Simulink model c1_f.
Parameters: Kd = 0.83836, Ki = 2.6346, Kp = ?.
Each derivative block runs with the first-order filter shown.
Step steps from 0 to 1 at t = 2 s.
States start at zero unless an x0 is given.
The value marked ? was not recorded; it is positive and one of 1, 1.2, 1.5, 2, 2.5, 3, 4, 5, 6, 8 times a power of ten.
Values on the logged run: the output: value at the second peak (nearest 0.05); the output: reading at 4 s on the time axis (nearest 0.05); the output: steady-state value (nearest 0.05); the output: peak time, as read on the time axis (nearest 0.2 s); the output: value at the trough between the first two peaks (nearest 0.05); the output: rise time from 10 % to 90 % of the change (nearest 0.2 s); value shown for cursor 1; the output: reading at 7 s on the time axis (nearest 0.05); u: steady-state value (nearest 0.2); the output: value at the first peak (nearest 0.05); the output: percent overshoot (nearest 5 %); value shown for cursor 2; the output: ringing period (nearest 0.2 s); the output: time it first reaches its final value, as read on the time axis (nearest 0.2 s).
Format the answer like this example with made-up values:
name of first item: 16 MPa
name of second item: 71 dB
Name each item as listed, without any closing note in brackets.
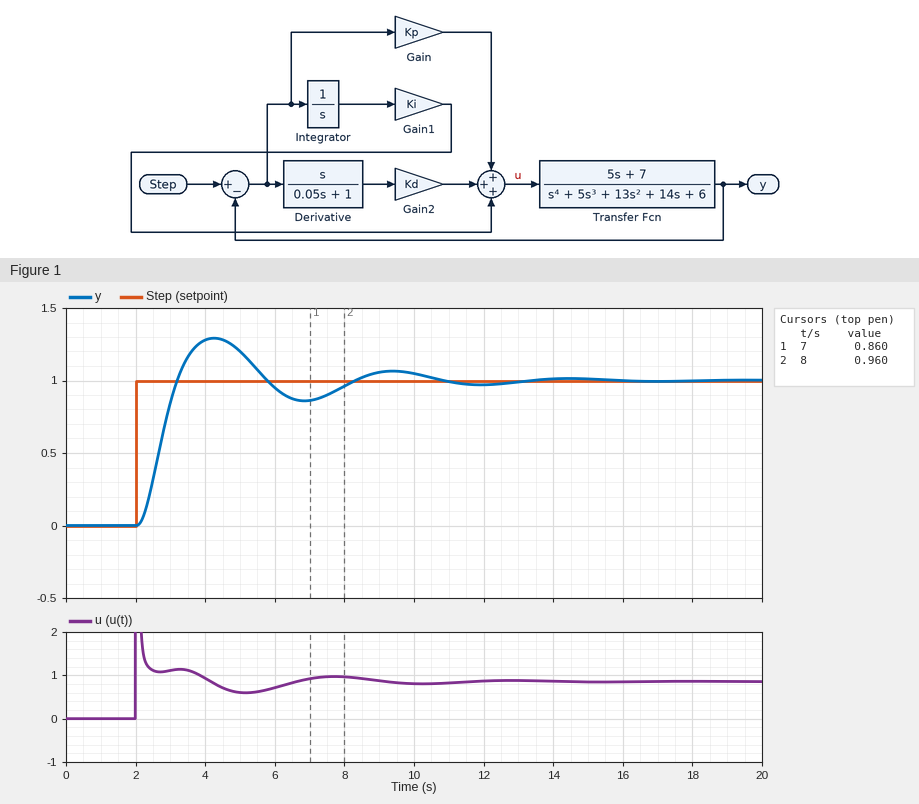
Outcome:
the output: value at the second peak: 1.05
the output: reading at 4 s on the time axis: 1.30
the output: steady-state value: 1.00
the output: peak time, as read on the time axis: 4.2 s
the output: value at the trough between the first two peaks: 0.85
the output: rise time from 10 % to 90 % of the change: 0.8 s
value shown for cursor 1: 0.860
the output: reading at 7 s on the time axis: 0.85
u: steady-state value: 0.8
the output: value at the first peak: 1.30
the output: percent overshoot: 30 %
value shown for cursor 2: 0.960
the output: ringing period: 5.2 s
the output: time it first reaches its final value, as read on the time axis: 3.2 s
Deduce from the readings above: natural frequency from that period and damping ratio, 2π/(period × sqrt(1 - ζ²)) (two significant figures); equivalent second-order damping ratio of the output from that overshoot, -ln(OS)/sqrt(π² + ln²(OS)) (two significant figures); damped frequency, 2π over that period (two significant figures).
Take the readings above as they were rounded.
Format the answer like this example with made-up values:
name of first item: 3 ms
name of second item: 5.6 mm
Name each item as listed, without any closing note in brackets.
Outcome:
natural frequency from that period and damping ratio, 2π/(period × sqrt(1 - ζ²)): 1.3 rad/s
equivalent second-order damping ratio of the output from that overshoot, -ln(OS)/sqrt(π² + ln²(OS)): 0.36
damped frequency, 2π over that period: 1.2 rad/s
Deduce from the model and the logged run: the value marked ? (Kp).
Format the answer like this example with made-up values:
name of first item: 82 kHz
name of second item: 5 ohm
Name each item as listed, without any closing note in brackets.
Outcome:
the value marked ?: 1.2
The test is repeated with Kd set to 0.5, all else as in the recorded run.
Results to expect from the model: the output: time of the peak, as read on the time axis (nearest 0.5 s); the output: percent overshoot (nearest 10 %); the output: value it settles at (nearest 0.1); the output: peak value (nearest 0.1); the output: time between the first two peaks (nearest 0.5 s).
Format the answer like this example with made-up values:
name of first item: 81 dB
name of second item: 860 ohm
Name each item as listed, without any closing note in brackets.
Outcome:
the output: time of the peak, as read on the time axis: 4.0 s
the output: percent overshoot: 50 %
the output: value it settles at: 1.0
the output: peak value: 1.5
the output: time between the first two peaks: 4.5 s
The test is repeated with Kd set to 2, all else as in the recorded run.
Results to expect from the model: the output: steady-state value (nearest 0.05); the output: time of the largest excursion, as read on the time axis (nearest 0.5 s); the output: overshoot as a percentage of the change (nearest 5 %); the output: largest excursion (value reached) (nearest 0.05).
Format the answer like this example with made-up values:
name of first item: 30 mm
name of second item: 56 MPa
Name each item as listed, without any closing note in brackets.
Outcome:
the output: steady-state value: 1.00
the output: time of the largest excursion, as read on the time axis: 5.0 s
the output: overshoot as a percentage of the change: 15 %
the output: largest excursion (value reached): 1.15
